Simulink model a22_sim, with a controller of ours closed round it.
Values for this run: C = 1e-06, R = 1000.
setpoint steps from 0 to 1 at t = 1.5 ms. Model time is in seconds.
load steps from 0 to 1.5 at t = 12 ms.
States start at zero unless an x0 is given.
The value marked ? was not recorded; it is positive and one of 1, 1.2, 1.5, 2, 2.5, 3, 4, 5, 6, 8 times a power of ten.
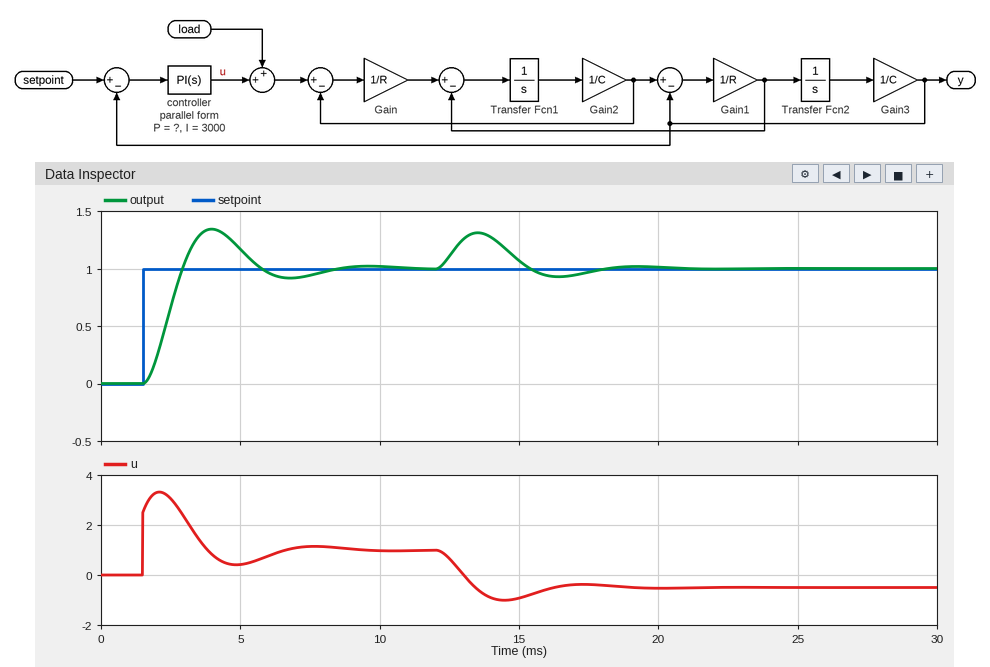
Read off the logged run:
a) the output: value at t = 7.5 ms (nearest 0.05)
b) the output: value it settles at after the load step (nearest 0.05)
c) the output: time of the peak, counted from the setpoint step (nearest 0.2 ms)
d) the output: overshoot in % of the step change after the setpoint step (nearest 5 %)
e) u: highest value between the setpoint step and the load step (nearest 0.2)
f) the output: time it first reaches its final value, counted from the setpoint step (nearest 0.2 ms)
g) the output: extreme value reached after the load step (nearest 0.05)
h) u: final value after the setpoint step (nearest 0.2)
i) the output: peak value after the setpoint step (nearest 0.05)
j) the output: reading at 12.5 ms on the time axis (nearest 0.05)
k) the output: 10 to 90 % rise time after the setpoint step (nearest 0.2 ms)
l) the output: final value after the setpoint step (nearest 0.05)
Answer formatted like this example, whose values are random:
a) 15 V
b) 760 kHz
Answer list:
a) 0.95
b) 1.00
c) 2.4 ms
d) 35 %
e) 3.4
f) 1.4 ms
g) 1.30
h) 1.0
i) 1.35
j) 1.10
k) 1.0 ms
l) 1.00
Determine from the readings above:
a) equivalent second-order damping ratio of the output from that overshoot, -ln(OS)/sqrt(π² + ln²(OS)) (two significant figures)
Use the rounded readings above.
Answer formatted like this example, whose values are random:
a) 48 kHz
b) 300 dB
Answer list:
a) 0.32
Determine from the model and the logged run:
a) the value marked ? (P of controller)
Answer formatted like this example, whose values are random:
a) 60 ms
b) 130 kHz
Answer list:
a) 2.5
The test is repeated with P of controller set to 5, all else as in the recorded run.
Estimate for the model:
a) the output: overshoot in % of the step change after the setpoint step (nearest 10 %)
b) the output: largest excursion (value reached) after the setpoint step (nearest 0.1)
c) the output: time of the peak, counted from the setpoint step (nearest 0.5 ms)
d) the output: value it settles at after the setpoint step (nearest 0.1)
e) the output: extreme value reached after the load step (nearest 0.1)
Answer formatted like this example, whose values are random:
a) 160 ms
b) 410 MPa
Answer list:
a) 20 %
b) 1.2
c) 1.5 ms
d) 1.0
e) 1.2
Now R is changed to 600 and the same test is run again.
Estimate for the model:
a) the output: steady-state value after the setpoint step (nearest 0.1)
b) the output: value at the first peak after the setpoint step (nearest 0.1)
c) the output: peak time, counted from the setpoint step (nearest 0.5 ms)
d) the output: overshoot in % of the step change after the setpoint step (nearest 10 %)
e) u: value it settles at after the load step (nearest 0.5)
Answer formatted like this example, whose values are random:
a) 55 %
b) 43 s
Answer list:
a) 1.0
b) 1.2
c) 1.5 ms
d) 20 %
e) -0.5
